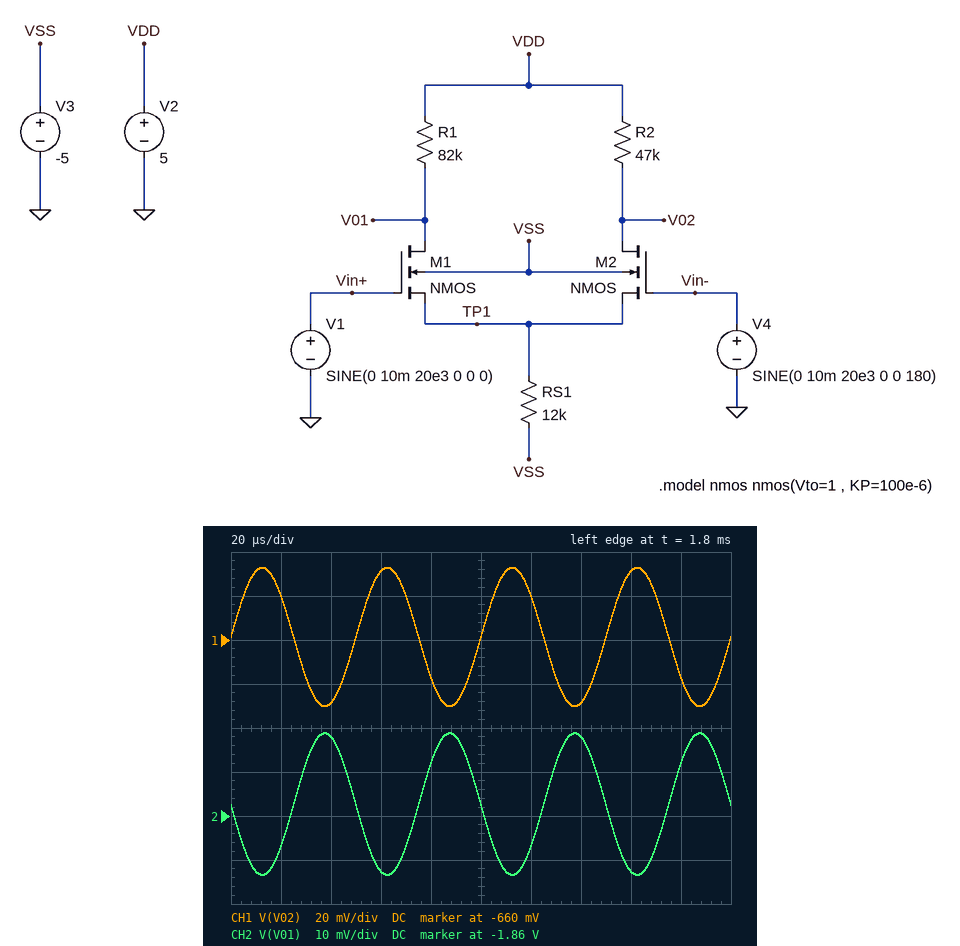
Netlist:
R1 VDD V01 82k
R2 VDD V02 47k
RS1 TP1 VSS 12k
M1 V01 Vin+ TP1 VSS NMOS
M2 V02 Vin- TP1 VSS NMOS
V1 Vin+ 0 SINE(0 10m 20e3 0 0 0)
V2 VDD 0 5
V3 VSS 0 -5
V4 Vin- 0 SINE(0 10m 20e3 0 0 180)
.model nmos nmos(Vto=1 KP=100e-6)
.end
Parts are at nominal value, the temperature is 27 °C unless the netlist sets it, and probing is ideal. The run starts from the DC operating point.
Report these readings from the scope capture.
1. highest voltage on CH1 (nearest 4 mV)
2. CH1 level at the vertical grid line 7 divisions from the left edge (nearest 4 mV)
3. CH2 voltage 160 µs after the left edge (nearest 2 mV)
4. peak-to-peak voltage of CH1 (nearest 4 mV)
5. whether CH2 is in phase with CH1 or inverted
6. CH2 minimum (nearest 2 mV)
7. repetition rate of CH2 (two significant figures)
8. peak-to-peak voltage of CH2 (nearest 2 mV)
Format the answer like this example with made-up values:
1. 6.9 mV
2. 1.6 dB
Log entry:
1. -628 mV
2. -688 mV
3. -1.872 V
4. 64 mV
5. inverted
6. -1.874 V
7. 20 kHz
8. 32 mV
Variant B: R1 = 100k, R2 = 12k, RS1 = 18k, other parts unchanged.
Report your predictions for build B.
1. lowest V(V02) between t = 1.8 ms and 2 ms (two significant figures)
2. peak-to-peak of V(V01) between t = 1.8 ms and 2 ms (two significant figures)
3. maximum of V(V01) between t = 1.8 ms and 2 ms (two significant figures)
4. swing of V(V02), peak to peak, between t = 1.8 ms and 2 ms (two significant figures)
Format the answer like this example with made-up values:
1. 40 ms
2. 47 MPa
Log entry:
1. 4.0 V
2. 42 mV
3. -1.6 V
4. 13 mV
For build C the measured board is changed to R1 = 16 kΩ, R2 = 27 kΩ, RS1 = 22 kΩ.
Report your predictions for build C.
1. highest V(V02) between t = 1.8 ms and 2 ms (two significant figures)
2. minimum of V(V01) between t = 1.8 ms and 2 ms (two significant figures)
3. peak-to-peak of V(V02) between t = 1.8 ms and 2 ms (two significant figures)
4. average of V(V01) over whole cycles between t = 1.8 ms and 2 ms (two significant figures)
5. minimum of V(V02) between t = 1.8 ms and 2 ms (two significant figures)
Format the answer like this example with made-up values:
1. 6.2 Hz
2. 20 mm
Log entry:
1. 3.3 V
2. 3.9 V
3. 62 mV
4. 4.0 V
5. 3.2 V
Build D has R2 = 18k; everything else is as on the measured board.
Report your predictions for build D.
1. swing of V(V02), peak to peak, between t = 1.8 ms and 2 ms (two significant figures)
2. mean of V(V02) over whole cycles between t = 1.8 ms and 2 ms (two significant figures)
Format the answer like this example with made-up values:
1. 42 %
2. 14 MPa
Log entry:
1. 24 mV
2. 2.8 V
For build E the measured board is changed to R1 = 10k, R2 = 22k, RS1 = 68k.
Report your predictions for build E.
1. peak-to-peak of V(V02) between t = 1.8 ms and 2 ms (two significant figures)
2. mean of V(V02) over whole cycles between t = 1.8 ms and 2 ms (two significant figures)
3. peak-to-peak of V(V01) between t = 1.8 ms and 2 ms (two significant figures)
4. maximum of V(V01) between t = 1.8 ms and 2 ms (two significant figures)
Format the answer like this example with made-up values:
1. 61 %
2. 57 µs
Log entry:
1. 31 mV
2. 4.5 V
3. 14 mV
4. 4.8 V
